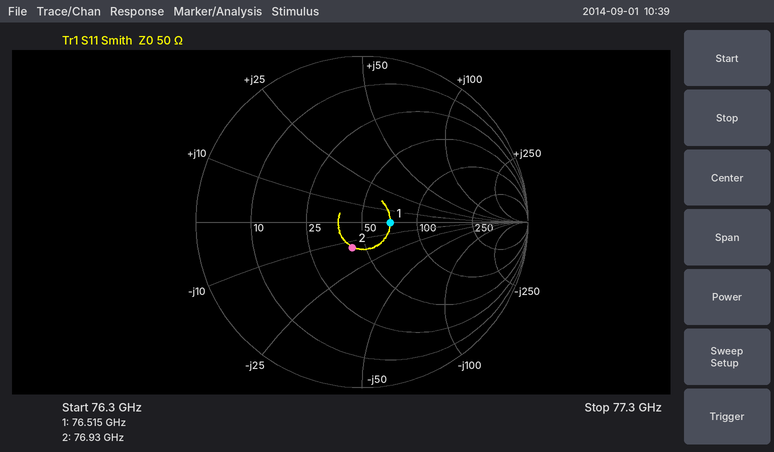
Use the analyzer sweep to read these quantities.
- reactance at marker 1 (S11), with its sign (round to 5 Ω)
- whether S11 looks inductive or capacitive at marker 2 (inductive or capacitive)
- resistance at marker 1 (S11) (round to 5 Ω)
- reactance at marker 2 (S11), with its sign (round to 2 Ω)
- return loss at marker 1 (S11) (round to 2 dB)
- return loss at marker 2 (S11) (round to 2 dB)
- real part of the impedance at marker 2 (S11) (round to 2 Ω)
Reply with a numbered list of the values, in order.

1. 0 Ω
2. capacitive
3. 70 Ω
4. -14 Ω
5. 16 dB
6. 16 dB
7. 42 Ω
